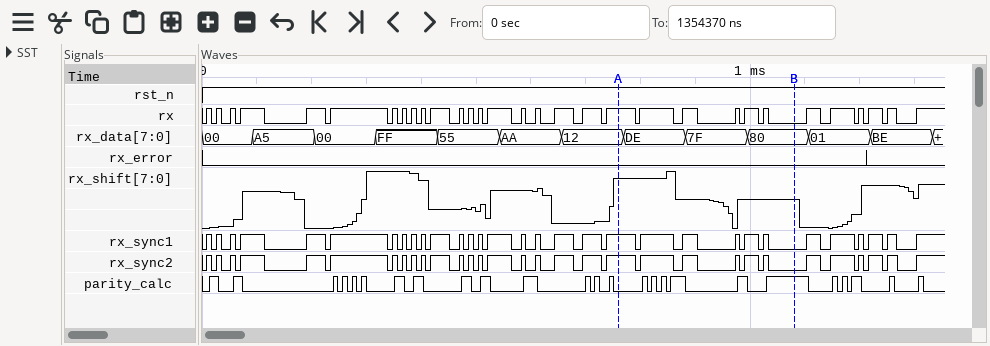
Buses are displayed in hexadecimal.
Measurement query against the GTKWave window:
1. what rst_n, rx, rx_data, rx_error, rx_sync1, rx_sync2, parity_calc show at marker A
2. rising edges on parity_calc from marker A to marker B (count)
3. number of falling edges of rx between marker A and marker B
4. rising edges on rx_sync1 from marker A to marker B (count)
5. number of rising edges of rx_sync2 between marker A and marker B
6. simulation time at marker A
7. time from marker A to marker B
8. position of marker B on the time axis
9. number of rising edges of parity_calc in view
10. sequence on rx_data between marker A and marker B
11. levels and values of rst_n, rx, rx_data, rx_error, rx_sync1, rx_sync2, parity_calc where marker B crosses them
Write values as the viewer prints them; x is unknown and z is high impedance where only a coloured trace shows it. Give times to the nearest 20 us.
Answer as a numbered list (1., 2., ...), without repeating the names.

1. rst_n=1, rx=1, rx_data=12, rx_error=0, rx_sync1=1, rx_sync2=1, parity_calc=0
2. 6
3. 6
4. 5
5. 5
6. 760 us
7. 320 us
8. 1080 us
9. 25
10. 12, DE, 7F, 80
11. rst_n=1, rx=0, rx_data=80, rx_error=0, rx_sync1=0, rx_sync2=0, parity_calc=1
